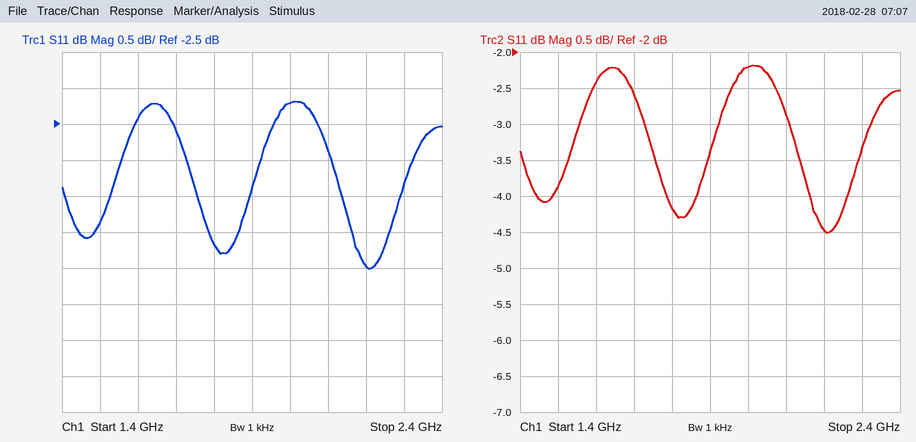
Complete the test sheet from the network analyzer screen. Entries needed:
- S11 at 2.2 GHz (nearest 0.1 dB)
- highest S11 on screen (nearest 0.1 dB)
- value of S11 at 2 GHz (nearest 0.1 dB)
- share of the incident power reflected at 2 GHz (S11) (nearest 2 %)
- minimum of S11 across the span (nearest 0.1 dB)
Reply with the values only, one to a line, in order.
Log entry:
-4.5 dB
-2.2 dB
-2.2 dB
60 %
-4.5 dB
